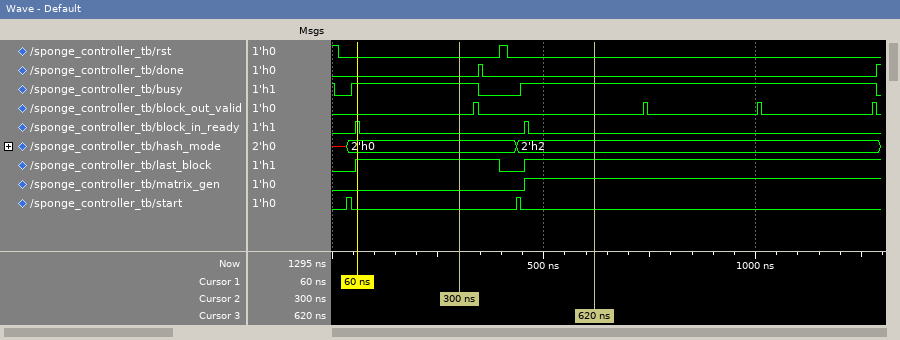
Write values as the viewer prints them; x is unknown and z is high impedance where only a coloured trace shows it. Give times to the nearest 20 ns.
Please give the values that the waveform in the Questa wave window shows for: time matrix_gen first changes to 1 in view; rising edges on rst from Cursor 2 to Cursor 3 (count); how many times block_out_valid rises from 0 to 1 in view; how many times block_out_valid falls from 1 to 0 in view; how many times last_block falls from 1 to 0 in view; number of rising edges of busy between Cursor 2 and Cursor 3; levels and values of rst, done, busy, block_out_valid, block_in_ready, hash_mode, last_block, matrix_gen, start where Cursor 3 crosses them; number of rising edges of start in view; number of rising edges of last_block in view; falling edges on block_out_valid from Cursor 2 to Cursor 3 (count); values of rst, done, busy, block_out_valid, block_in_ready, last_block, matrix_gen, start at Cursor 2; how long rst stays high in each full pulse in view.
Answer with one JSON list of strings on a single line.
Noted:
["460 ns", "1", "4", "4", "1", "1", "rst=0, done=0, busy=1, block_out_valid=0, block_in_ready=0, hash_mode=2'h2, last_block=1, matrix_gen=1, start=0", "2", "2", "1", "rst=0, done=0, busy=1, block_out_valid=0, block_in_ready=0, last_block=1, matrix_gen=0, start=0", "20 ns"]
